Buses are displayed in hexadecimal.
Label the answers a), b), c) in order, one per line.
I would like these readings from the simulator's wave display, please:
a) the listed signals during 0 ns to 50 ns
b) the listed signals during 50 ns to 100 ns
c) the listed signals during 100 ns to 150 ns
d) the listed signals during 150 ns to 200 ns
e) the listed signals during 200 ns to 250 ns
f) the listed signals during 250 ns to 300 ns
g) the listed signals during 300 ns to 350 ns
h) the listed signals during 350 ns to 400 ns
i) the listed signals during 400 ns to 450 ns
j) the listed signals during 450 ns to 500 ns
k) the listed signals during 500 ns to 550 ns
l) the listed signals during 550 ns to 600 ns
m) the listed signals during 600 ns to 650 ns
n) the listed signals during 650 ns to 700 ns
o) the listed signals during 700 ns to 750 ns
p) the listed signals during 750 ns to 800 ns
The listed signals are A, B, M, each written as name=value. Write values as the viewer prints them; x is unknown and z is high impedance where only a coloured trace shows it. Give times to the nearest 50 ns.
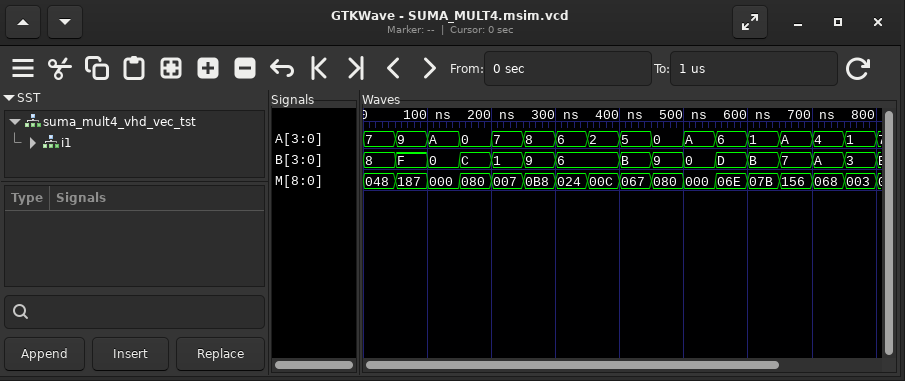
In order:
a) A=7, B=8, M=048
b) A=9, B=F, M=187
c) A=A, B=0, M=000
d) A=0, B=C, M=080
e) A=7, B=1, M=007
f) A=8, B=9, M=0B8
g) A=6, B=6, M=024
h) A=2, B=6, M=00C
i) A=5, B=B, M=067
j) A=0, B=9, M=080
k) A=A, B=0, M=000
l) A=6, B=D, M=06E
m) A=1, B=B, M=07B
n) A=A, B=7, M=156
o) A=4, B=A, M=068
p) A=1, B=3, M=003
